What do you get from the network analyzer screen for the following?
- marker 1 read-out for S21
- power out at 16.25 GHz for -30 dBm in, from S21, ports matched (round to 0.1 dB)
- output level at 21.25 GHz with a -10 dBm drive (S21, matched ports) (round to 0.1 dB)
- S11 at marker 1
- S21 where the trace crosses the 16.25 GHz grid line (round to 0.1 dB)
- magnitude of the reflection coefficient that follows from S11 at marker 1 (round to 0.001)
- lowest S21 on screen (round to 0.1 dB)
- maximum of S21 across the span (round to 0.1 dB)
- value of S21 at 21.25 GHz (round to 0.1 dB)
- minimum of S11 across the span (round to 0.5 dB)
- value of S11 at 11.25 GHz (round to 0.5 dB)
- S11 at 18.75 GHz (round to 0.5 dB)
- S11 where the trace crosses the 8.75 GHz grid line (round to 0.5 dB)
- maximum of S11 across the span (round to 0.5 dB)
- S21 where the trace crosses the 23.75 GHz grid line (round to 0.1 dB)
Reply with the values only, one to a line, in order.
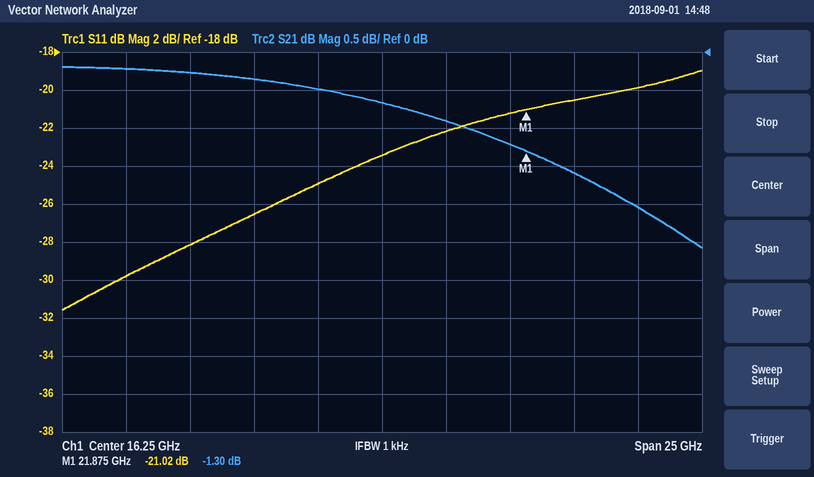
-1.30 dB
-30.7 dBm
-11.2 dBm
-21.02 dB
-0.7 dB
0.089
-2.6 dB
-0.2 dB
-1.2 dB
-31.5 dB
-26.5 dB
-22.0 dB
-28.0 dB
-19.0 dB
-1.6 dB
